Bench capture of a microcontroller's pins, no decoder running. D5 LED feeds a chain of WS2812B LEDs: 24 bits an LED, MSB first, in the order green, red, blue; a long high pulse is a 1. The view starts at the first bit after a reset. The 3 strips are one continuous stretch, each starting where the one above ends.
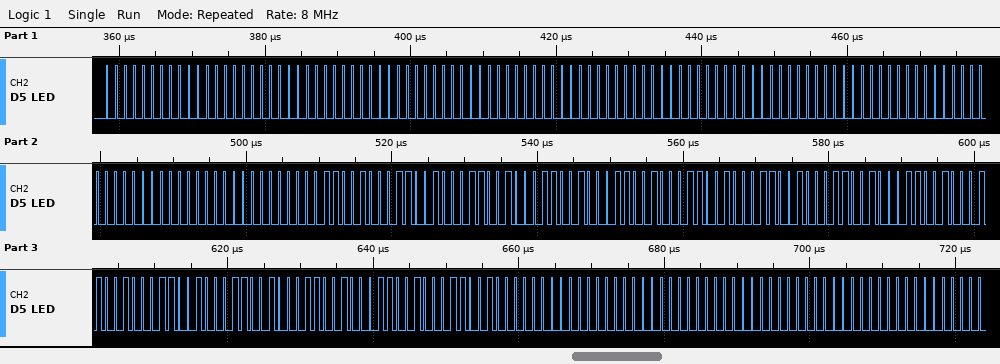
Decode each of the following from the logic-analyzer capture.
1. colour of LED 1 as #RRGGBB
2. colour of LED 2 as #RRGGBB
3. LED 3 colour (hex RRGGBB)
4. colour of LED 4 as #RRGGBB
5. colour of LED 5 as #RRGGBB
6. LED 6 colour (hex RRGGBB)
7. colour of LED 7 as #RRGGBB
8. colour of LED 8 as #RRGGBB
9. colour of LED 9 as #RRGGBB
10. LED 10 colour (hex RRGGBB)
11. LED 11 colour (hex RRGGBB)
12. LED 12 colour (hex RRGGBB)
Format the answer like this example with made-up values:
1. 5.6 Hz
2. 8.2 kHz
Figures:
1. #000000
2. #000000
3. #000000
4. #000000
5. #000000
6. #323232
7. #323232
8. #323232
9. #323232
10. #323232
11. #000000
12. #000000
